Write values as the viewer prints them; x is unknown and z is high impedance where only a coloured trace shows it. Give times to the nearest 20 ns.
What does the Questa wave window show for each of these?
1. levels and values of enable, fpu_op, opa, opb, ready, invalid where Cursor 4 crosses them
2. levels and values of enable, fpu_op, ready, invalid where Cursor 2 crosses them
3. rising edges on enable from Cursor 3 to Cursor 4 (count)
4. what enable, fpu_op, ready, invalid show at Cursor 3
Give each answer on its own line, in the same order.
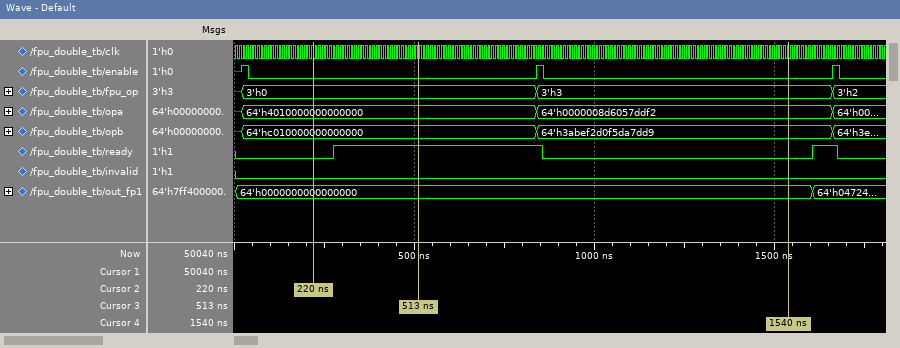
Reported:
enable=0, fpu_op=3'h3, opa=64'h0000008d6057ddf2, opb=64'h3abef2d0f5da7dd9, ready=0, invalid=0
enable=0, fpu_op=3'h0, ready=0, invalid=0
1
enable=0, fpu_op=3'h0, ready=1, invalid=0
